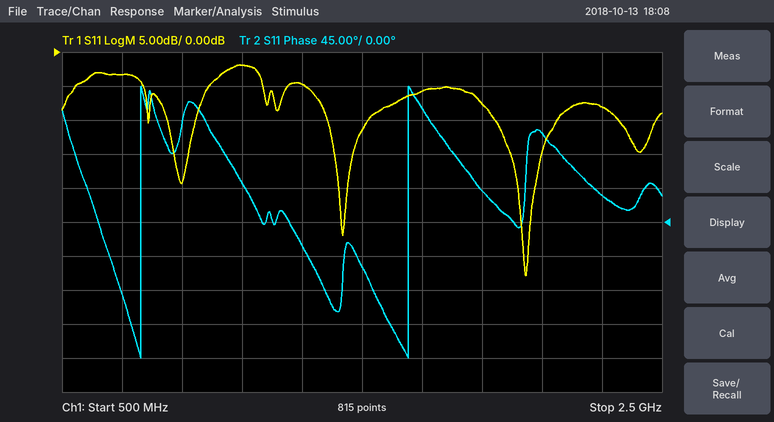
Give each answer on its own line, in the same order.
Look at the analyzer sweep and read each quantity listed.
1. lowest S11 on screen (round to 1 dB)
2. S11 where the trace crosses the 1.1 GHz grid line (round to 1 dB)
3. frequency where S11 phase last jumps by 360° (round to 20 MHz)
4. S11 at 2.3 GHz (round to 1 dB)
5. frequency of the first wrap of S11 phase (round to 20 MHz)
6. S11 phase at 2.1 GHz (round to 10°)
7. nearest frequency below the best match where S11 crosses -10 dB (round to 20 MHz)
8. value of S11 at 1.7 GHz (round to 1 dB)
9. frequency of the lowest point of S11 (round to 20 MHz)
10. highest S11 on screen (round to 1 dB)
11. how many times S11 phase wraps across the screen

-33 dB
-2 dB
1.66 GHz
-8 dB
760 MHz
120°
1.94 GHz
-6 dB
2.04 GHz
-2 dB
2
